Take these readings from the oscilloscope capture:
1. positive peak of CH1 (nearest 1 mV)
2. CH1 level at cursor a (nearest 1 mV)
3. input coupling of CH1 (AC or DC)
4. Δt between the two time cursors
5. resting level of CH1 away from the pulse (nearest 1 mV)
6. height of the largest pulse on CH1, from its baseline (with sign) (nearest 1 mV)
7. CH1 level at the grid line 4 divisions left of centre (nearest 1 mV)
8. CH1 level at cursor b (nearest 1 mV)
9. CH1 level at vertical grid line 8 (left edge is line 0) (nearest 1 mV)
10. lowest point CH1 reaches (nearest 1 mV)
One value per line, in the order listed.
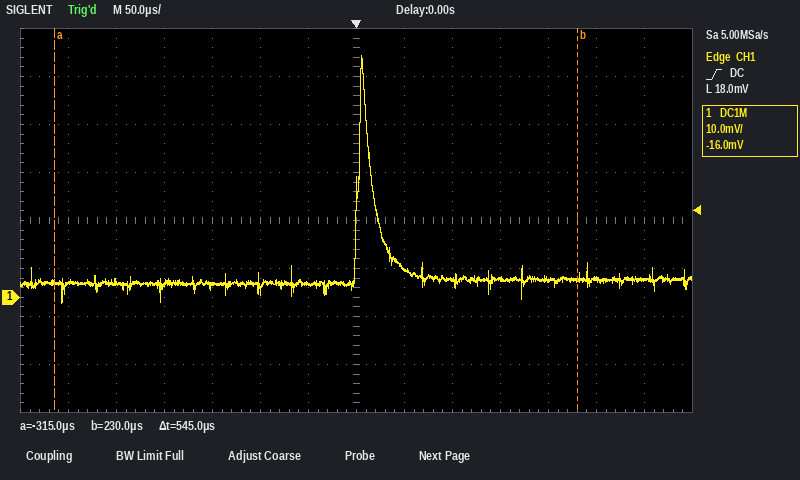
50 mV
3 mV
DC
545 µs
3 mV
+47 mV
3 mV
4 mV
6 mV
-1 mV
